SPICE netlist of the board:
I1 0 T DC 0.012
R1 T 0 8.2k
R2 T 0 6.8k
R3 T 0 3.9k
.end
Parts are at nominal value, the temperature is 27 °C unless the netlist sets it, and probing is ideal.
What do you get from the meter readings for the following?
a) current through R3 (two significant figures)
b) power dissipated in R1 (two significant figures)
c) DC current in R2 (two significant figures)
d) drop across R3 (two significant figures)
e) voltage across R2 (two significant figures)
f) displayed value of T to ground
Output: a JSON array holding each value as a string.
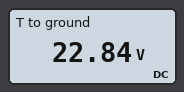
["5.9 mA", "64 mW", "3.4 mA", "23 V", "23 V", "22.84 V"]
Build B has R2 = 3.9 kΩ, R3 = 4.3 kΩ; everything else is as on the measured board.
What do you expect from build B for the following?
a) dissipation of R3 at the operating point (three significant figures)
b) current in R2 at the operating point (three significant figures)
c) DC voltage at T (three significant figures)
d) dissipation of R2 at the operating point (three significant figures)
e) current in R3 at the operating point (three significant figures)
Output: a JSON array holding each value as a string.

["89.7 mW", "5.04 mA", "19.6 V", "98.9 mW", "4.57 mA"]
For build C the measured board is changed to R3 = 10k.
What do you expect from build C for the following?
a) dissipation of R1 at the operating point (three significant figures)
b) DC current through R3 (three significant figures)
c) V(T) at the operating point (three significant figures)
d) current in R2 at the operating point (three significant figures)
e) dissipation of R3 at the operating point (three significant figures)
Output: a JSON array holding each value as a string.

["129 mW", "3.25 mA", "32.5 V", "4.78 mA", "106 mW"]
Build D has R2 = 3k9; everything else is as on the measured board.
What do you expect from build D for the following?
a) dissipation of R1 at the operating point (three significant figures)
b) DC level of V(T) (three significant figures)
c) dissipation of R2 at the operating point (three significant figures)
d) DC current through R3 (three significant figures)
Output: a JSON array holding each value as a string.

["43.6 mW", "18.9 V", "91.6 mW", "4.85 mA"]
